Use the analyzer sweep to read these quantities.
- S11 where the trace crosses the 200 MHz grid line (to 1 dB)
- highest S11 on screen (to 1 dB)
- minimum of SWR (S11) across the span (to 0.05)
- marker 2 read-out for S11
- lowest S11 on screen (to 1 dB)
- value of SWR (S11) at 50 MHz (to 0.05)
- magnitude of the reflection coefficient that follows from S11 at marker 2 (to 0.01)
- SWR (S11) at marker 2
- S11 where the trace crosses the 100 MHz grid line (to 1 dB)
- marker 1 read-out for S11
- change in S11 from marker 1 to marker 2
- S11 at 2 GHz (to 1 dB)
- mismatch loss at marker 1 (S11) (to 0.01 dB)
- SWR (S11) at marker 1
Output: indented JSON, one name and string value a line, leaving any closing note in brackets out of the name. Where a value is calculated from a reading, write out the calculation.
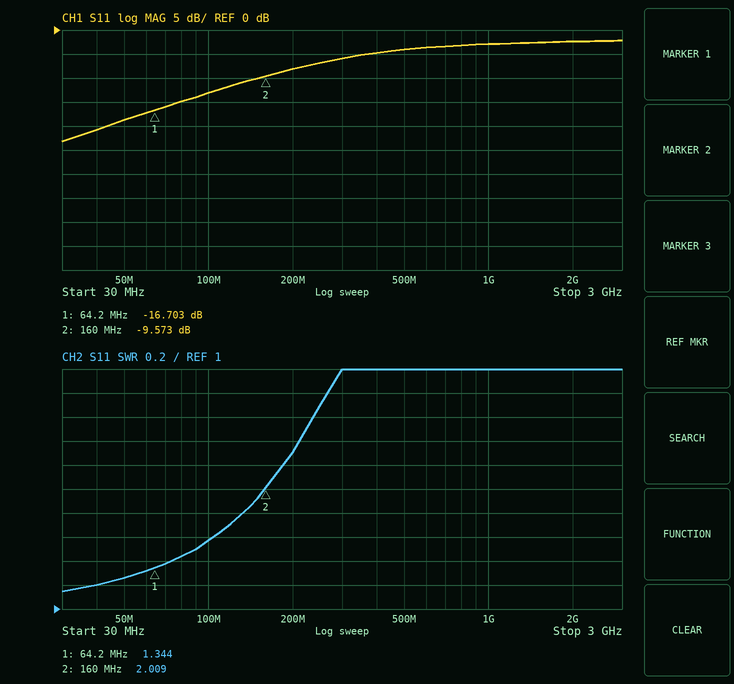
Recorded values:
{
  "S11 where the trace crosses the 200 MHz grid line": "-8 dB",
  "highest S11 on screen": "-2 dB",
  "minimum of SWR (S11) across the span": "1.15",
  "marker 2 read-out for S11": "-9.573 dB",
  "lowest S11 on screen": "-23 dB",
  "value of SWR (S11) at 50 MHz": "1.25",
  "magnitude of the reflection coefficient that follows from S11 at marker 2": "10^(-9.573/20) ≈ 0.33",
  "SWR (S11) at marker 2": "2.009",
  "S11 where the trace crosses the 100 MHz grid line": "-13 dB",
  "marker 1 read-out for S11": "-16.703 dB",
  "change in S11 from marker 1 to marker 2": "-9.573 − (-16.703) = 7.130 dB",
  "S11 at 2 GHz": "-2 dB",
  "mismatch loss at marker 1 (S11)": "−10 log10(1 − 10^(-16.703/10)) ≈ 0.09 dB",
  "SWR (S11) at marker 1": "1.344"
}
